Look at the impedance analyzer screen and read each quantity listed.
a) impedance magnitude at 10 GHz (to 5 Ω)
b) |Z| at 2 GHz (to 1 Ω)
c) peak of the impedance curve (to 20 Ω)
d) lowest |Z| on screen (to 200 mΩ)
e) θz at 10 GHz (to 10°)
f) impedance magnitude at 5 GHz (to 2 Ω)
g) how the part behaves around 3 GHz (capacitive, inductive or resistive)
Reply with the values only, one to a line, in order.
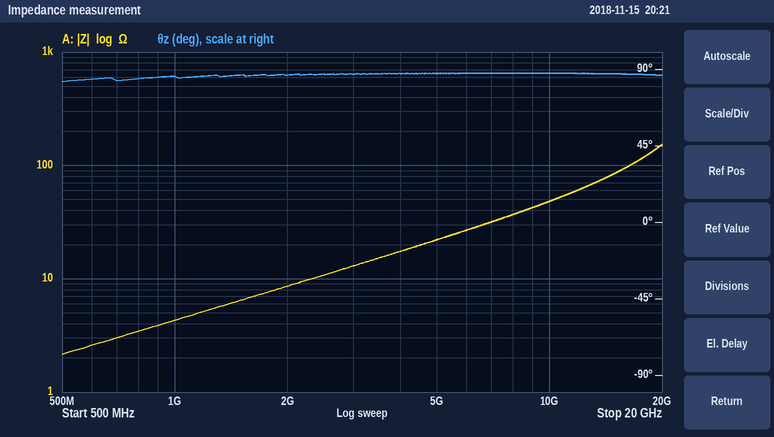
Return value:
50 Ω
9 Ω
160 Ω
2.2 Ω
90°
22 Ω
inductive
